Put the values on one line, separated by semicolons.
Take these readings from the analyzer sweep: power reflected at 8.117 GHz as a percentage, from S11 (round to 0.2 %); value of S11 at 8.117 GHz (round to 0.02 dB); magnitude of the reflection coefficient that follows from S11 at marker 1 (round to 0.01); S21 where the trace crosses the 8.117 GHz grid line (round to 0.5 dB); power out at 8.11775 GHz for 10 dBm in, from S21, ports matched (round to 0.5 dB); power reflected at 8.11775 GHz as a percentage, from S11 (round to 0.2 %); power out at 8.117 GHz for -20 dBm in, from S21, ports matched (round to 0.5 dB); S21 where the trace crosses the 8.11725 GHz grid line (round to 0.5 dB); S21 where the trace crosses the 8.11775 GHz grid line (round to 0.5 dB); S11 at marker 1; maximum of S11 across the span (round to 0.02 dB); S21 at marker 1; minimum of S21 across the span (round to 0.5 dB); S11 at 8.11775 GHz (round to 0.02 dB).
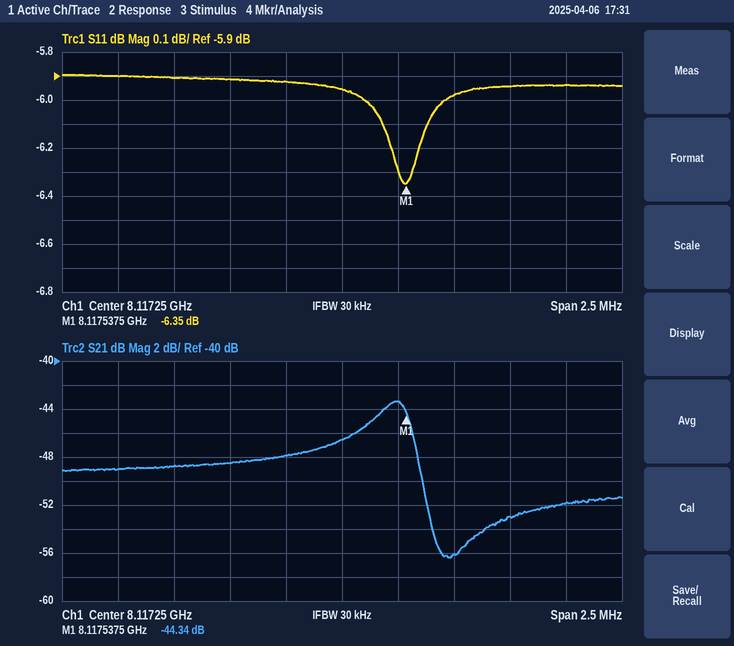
25.6 %; -5.92 dB; 0.48; -48.0 dB; -46.0 dBm; 25.2 %; -68.0 dBm; -46.5 dB; -56.0 dB; -6.35 dB; -5.90 dB; -44.34 dB; -56.5 dB; -5.98 dB
